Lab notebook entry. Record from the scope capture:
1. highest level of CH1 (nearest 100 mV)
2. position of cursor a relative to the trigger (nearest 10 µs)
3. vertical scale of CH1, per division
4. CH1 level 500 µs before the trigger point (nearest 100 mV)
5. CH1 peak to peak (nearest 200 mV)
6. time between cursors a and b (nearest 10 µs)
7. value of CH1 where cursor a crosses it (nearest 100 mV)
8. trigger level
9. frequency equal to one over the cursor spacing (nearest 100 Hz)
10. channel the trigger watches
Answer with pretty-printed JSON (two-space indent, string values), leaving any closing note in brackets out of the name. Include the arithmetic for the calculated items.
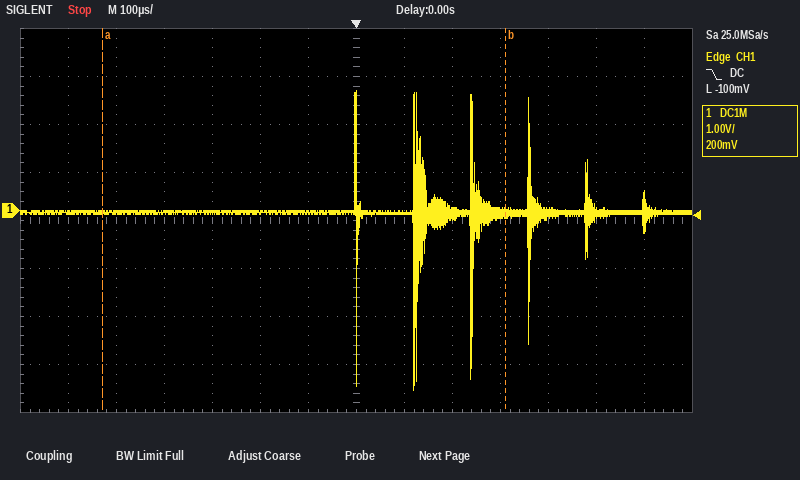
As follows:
{
  "highest level of CH1": "2.5 V",
  "position of cursor a relative to the trigger": "-530 µs",
  "vertical scale of CH1, per division": "1 V",
  "CH1 level 500 µs before the trigger point": "0.0 V",
  "CH1 peak to peak": "6.2 V",
  "time between cursors a and b": "840 µs",
  "value of CH1 where cursor a crosses it": "0.0 V",
  "trigger level": "-100 mV",
  "frequency equal to one over the cursor spacing": "1 / 840 µs ≈ 1.2 kHz",
  "channel the trigger watches": "CH1"
}
